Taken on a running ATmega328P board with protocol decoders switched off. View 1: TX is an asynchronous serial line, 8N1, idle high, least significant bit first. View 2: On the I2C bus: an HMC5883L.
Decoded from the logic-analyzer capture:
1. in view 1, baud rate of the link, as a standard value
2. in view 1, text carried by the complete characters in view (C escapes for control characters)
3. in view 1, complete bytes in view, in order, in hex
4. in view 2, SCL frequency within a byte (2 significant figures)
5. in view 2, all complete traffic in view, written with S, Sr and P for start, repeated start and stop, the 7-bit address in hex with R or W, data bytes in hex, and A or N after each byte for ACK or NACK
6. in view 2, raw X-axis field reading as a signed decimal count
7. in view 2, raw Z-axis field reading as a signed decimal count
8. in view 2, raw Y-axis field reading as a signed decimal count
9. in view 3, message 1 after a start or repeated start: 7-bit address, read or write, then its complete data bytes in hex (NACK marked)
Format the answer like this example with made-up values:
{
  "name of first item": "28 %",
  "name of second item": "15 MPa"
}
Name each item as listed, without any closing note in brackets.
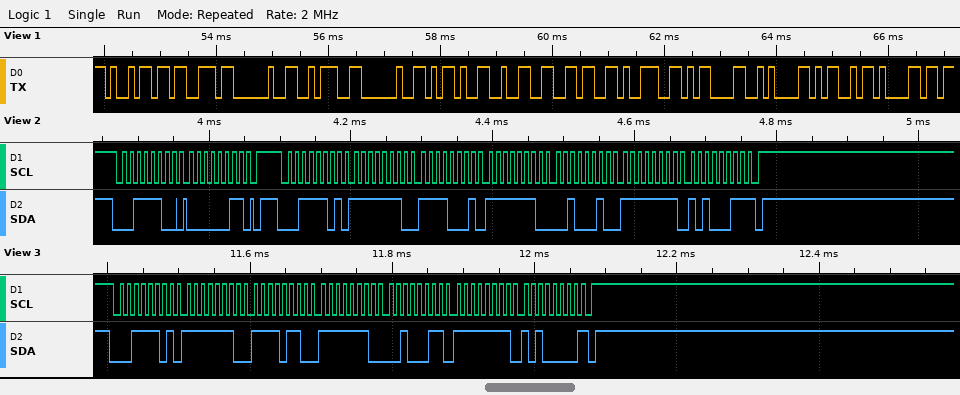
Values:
{
  "in view 1, baud rate of the link, as a standard value": "9600 baud",
  "in view 1, text carried by the complete characters in view": "\"is : -269\\r\\nMa\"",
  "in view 1, complete bytes in view, in order, in hex": "69 73 20 3A 20 2D 32 36 39 0D 0A 4D 61",
  "in view 2, SCL frequency within a byte": "100 kHz",
  "in view 2, all complete traffic in view, written with S, Sr and P for start, repeated start and stop, the 7-bit address in hex with R or W, data bytes in hex, and A or N after each byte for ACK or NACK": "S 1EW A 03 A P S 1ER A FE A F1 A FE A 22 A FF A A3 N P",
  "in view 2, raw X-axis field reading as a signed decimal count": "-271",
  "in view 2, raw Z-axis field reading as a signed decimal count": "-478",
  "in view 2, raw Y-axis field reading as a signed decimal count": "-93",
  "in view 3, message 1 after a start or repeated start: 7-bit address, read or write, then its complete data bytes in hex": "0x1E read: FE F6 FE 23 FF A0 NACK"
}
